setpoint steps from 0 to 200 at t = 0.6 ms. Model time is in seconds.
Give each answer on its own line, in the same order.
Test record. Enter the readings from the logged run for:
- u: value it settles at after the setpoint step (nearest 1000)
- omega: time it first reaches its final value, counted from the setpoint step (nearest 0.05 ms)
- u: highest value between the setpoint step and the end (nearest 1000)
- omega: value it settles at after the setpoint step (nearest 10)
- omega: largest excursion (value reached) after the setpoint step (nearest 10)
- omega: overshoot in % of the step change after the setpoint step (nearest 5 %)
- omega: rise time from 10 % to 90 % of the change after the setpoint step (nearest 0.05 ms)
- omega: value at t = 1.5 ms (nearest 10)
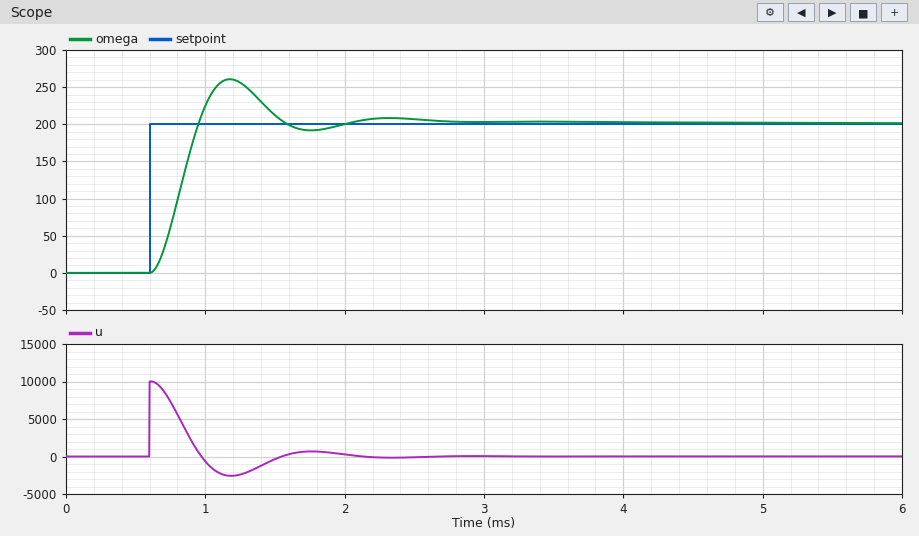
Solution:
0
0.35 ms
10000
200
260
30 %
0.25 ms
210
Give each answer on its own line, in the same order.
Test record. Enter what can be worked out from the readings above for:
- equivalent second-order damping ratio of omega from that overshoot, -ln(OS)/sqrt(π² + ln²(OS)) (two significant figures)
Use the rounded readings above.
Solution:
0.36
